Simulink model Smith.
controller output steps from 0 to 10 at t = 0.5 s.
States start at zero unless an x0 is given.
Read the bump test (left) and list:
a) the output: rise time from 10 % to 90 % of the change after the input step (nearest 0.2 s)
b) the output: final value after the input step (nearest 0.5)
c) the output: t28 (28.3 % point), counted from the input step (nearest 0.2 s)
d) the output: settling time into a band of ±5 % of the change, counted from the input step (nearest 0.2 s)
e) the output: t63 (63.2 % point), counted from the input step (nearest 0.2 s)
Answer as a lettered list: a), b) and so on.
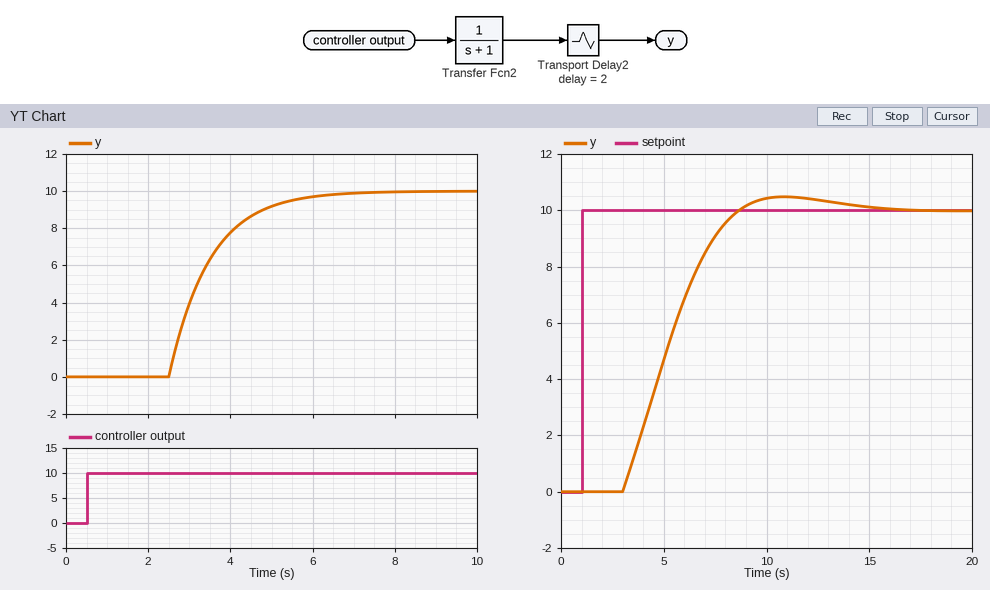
a) 2.2 s
b) 10.0
c) 2.4 s
d) 5.0 s
e) 3.0 s
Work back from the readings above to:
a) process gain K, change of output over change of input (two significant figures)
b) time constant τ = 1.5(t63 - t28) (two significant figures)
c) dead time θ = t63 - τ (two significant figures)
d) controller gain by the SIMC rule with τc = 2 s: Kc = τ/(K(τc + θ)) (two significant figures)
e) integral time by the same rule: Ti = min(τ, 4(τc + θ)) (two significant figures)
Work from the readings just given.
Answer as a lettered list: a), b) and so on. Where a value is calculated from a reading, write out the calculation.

a) (10 - 0) / 10 = 1.0
b) 1.5 × (3 - 2.4) = 0.90 s
c) 3 - 0.9 = 2.1 s
d) 0.9 / (1 × (2 + 2.1)) = 0.22
e) min(0.9, 4 × (2 + 2.1)) = 0.90 s
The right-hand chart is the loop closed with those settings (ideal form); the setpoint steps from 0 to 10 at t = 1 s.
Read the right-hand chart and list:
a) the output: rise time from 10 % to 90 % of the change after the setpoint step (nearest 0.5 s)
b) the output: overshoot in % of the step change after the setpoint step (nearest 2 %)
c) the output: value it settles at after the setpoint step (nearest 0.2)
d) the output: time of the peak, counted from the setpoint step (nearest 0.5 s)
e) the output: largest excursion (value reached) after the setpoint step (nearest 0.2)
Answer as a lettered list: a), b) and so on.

a) 4.0 s
b) 4 %
c) 10.0
d) 10.0 s
e) 10.4
